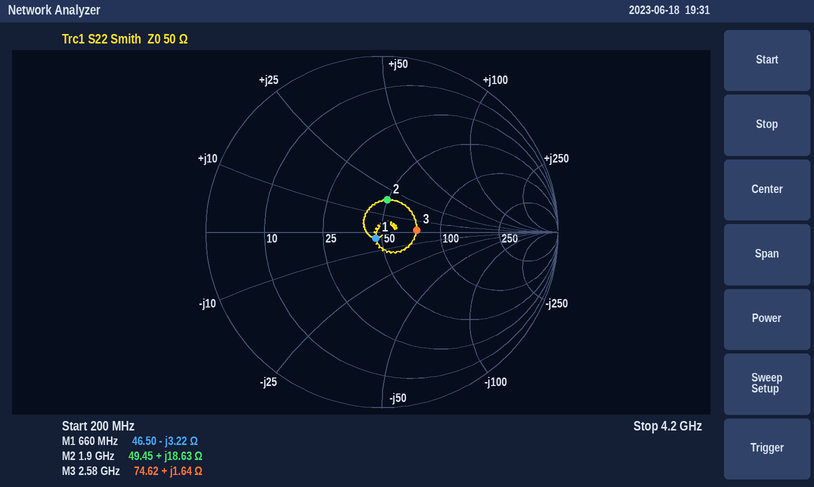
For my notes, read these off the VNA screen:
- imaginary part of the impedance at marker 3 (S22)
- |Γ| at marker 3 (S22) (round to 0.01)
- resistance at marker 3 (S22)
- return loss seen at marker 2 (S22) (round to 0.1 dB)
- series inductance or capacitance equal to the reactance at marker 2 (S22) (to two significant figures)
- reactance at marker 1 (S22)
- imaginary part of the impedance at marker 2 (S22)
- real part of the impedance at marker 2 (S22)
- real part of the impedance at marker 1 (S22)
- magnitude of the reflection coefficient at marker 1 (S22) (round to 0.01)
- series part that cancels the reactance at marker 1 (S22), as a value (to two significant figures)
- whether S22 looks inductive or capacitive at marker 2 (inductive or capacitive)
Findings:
+1.64 Ω
0.20
74.62 Ω
14.7 dB
1.6 nH
-3.22 Ω
+18.63 Ω
49.45 Ω
46.50 Ω
0.05
780 pH
inductive
